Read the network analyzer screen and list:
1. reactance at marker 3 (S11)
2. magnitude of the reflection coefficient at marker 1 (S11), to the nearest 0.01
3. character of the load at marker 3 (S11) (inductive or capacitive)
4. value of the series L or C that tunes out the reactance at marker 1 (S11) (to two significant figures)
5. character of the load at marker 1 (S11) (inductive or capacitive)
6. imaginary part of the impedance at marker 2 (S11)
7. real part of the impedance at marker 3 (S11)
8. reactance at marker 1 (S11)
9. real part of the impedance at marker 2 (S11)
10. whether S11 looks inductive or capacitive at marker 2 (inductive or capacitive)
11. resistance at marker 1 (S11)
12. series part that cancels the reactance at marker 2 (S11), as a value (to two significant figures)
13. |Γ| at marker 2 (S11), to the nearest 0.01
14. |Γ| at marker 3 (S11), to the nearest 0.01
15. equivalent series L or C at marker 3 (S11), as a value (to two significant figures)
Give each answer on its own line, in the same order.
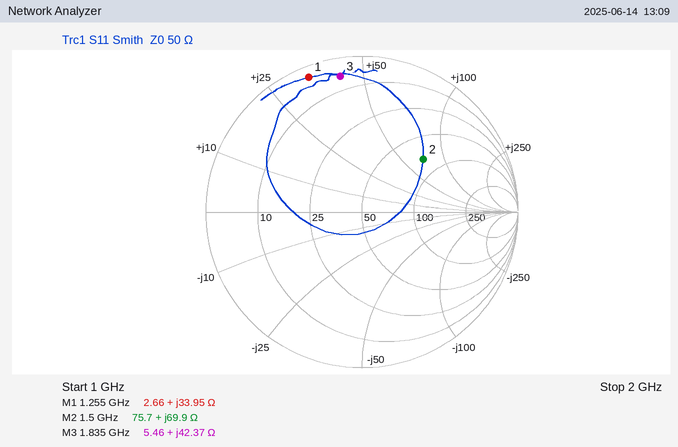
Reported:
+42.37 Ω
0.93
inductive
3.7 pF
inductive
+69.9 Ω
5.46 Ω
+33.95 Ω
75.7 Ω
inductive
2.66 Ω
1.5 pF
0.52
0.88
3.7 nH
